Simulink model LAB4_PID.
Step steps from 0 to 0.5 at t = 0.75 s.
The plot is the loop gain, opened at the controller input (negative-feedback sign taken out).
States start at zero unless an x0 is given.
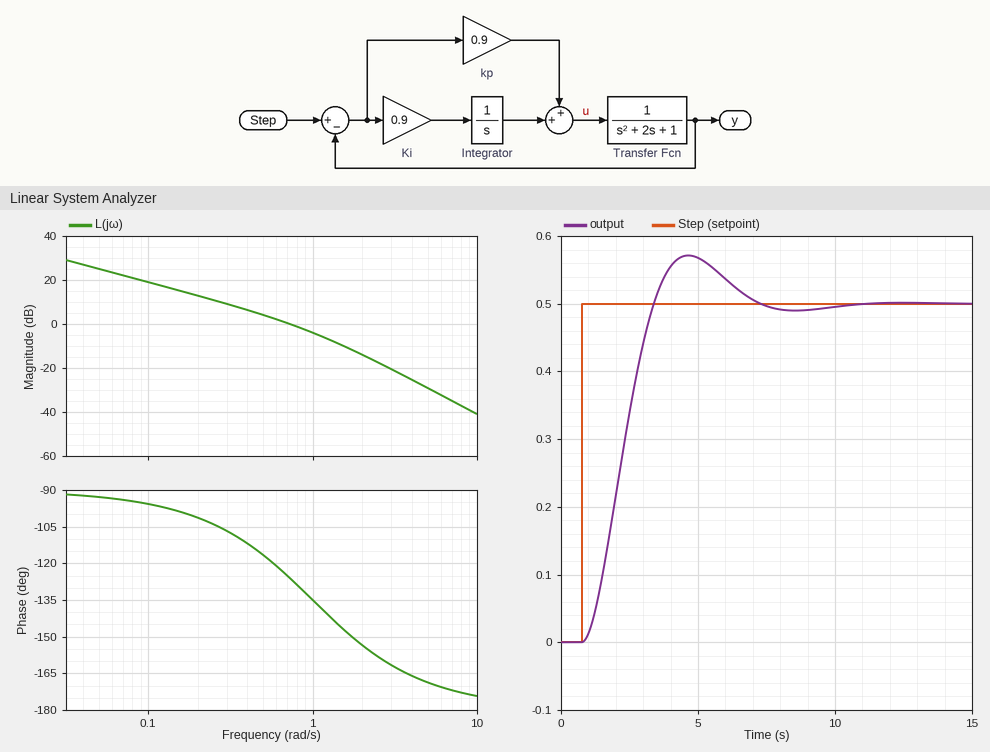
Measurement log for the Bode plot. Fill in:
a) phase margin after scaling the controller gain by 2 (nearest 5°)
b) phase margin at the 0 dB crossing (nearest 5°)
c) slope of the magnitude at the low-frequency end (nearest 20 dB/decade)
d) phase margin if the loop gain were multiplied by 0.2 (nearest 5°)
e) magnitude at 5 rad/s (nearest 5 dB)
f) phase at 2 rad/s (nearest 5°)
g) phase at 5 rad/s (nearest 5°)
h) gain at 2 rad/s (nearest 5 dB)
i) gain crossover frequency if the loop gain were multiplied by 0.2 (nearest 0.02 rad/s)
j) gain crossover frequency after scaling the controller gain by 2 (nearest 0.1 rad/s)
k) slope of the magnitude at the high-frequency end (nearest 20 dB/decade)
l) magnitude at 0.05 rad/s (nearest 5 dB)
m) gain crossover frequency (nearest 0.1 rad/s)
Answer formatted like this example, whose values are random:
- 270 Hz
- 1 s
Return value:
- 40°
- 55°
- -20 dB/decade
- 80°
- -30 dB
- -155°
- -170°
- -15 dB
- 0.18 rad/s
- 1.2 rad/s
- -40 dB/decade
- 25 dB
- 0.7 rad/s
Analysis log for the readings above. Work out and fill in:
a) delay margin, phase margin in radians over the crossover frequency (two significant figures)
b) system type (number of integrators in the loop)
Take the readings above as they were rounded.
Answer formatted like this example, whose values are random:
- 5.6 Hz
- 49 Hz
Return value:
- 1.4 s
- 1
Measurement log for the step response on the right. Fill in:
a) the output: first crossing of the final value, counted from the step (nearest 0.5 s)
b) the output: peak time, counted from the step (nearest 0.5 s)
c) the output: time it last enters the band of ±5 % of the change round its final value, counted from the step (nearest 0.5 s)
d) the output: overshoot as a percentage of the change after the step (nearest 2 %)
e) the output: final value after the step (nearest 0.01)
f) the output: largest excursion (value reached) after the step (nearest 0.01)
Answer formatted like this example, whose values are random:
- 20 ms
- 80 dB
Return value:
- 2.5 s
- 4.0 s
- 5.5 s
- 14 %
- 0.50
- 0.57
